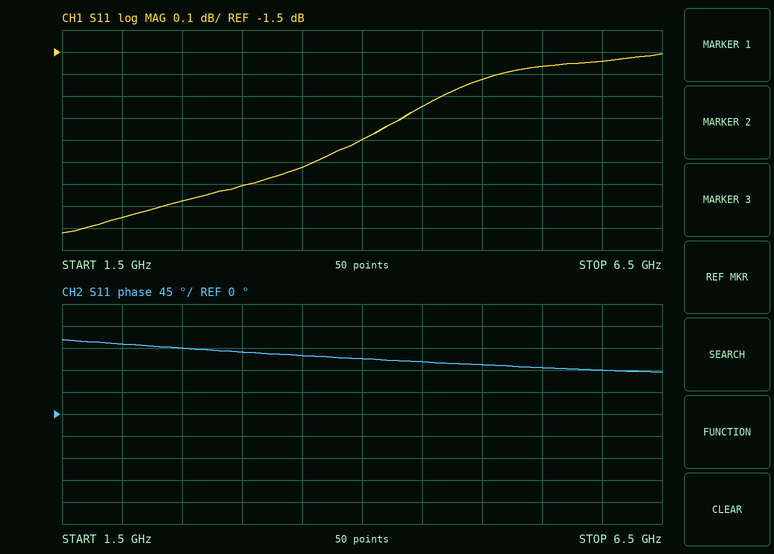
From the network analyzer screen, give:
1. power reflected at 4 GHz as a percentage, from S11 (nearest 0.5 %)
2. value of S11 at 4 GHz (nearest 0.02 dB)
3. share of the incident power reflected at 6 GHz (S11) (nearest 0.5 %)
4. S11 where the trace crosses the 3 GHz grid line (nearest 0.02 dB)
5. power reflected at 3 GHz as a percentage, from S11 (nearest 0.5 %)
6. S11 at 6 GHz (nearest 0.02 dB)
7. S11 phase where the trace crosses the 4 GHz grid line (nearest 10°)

64.5 %
-1.90 dB
70.0 %
-2.10 dB
61.5 %
-1.54 dB
110°
